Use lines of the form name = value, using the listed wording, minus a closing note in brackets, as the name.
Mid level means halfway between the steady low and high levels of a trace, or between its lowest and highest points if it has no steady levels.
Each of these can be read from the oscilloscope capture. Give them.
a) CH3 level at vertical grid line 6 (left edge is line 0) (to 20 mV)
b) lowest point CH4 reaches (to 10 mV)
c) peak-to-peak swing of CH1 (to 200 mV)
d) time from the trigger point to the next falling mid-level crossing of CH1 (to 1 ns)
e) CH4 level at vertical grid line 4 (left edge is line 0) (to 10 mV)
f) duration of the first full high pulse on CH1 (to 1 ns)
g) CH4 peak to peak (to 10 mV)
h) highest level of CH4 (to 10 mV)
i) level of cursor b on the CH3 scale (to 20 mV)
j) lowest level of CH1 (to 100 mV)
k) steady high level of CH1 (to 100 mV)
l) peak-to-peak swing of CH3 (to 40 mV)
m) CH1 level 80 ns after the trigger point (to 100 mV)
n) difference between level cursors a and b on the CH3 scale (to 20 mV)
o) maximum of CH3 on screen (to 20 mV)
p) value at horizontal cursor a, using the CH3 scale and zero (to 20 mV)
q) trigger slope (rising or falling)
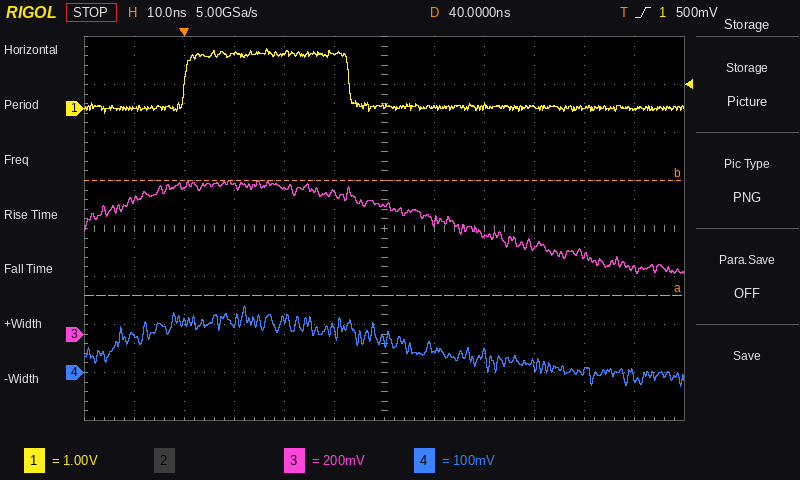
CH3 level at vertical grid line 6 (left edge is line 0) = 540 mV
lowest point CH4 reaches = -30 mV
peak-to-peak swing of CH1 = 1.4 V
time from the trigger point to the next falling mid-level crossing of CH1 = 33 ns
CH4 level at vertical grid line 4 (left edge is line 0) = 110 mV
duration of the first full high pulse on CH1 = 33 ns
CH4 peak to peak = 170 mV
highest level of CH4 = 140 mV
level of cursor b on the CH3 scale = 640 mV
lowest level of CH1 = -100 mV
steady high level of CH1 = 1.1 V
peak-to-peak swing of CH3 = 400 mV
CH1 level 80 ns after the trigger point = 0.0 V
difference between level cursors a and b on the CH3 scale = 480 mV
maximum of CH3 on screen = 640 mV
value at horizontal cursor a, using the CH3 scale and zero = 160 mV
trigger slope = rising
